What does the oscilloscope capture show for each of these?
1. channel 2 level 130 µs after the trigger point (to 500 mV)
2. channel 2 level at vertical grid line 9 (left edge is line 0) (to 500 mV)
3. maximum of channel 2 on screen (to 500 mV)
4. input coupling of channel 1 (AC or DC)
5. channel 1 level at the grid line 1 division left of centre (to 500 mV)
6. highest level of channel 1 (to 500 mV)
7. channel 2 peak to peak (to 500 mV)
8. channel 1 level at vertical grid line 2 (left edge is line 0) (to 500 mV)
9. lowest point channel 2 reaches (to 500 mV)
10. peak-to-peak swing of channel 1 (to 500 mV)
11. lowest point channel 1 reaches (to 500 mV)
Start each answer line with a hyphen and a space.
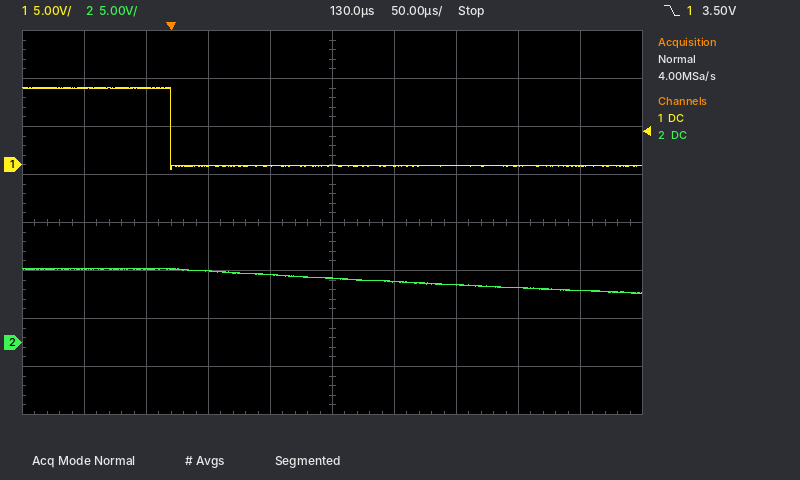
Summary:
- 6.5 V
- 5.5 V
- 7.5 V
- DC
- 0.0 V
- 8.0 V
- 2.5 V
- 8.0 V
- 5.0 V
- 8.5 V
- -500 mV
